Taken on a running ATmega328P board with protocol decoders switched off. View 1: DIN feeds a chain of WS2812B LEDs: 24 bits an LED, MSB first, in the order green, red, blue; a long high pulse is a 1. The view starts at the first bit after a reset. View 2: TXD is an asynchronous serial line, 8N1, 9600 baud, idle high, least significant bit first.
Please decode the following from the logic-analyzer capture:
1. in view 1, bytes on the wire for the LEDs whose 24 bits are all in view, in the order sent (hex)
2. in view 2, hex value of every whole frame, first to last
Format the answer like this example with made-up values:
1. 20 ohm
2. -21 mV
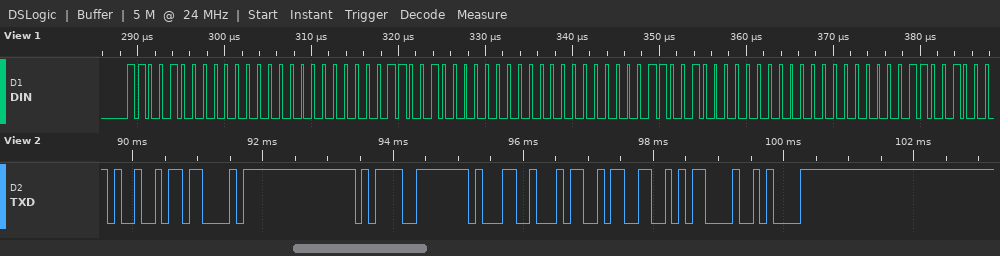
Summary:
1. C8 00 00 C8 00 00 C8 00 00
2. 49 43 3D 31 34 33 0D 0A
